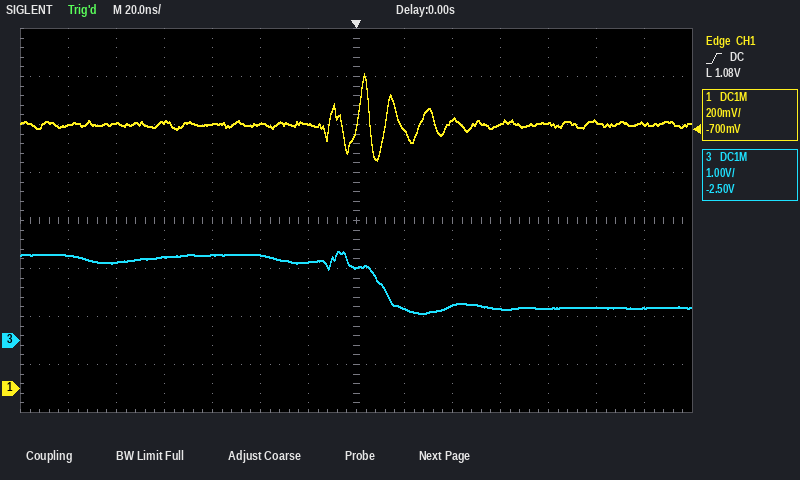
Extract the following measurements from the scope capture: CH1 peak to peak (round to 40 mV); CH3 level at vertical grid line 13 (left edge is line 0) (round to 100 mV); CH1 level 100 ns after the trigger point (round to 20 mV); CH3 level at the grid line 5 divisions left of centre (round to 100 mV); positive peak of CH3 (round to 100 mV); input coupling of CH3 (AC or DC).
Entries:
360 mV
700 mV
1.12 V
1.6 V
1.9 V
DC
